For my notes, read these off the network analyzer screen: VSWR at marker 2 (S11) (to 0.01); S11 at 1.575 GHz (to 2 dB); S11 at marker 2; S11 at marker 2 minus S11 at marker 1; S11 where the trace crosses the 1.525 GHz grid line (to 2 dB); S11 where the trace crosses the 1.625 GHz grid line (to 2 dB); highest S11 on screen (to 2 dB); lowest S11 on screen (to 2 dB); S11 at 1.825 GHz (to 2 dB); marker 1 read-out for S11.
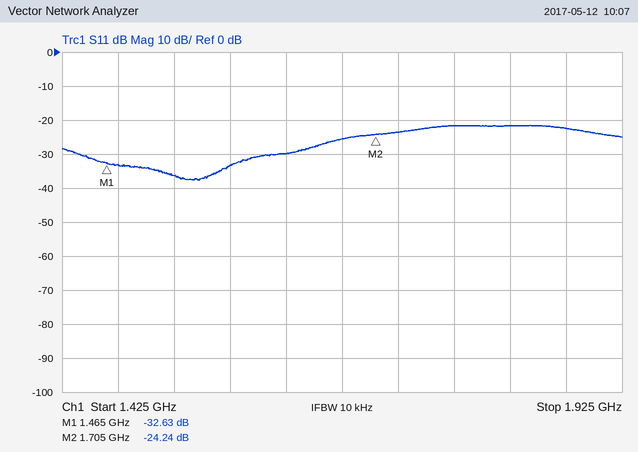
1.13
-34 dB
-24.24 dB
8.39 dB
-36 dB
-30 dB
-22 dB
-38 dB
-22 dB
-32.63 dB
